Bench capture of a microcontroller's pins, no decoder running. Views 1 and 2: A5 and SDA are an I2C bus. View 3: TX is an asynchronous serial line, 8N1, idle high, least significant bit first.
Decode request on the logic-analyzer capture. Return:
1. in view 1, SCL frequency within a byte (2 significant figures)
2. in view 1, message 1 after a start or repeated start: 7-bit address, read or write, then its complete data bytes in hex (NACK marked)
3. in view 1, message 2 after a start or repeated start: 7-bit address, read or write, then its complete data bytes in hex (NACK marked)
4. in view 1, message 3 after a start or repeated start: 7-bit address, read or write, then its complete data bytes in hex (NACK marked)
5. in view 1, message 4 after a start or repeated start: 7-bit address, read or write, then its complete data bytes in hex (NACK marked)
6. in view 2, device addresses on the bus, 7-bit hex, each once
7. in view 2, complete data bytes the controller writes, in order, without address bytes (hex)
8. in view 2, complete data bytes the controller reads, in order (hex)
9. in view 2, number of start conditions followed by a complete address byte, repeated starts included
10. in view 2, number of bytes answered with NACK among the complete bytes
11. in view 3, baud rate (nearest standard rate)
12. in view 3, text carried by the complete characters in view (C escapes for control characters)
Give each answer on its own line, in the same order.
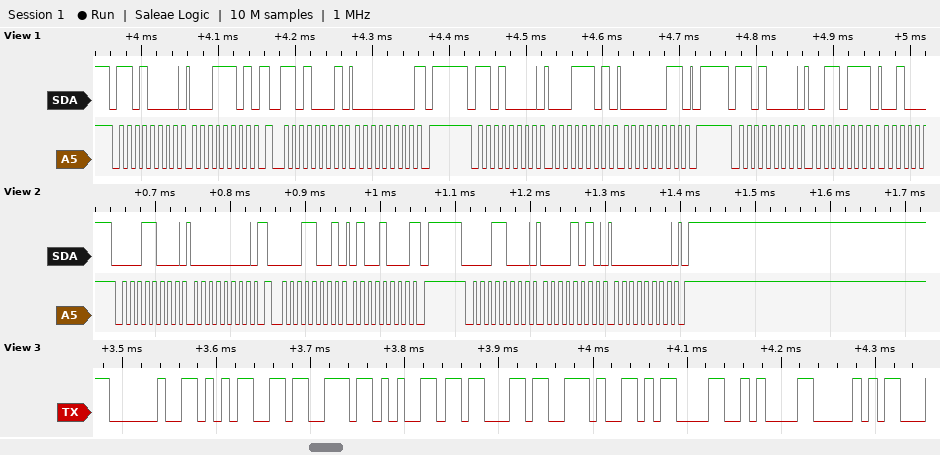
100 kHz
0x68 write: 1D
0x68 read: 00 NACK
0x68 write: 1D 03
0x68 write: 37
0x0C
00 0A 00
48
3
1
115200 baud
" 5sec.\r\nP"
